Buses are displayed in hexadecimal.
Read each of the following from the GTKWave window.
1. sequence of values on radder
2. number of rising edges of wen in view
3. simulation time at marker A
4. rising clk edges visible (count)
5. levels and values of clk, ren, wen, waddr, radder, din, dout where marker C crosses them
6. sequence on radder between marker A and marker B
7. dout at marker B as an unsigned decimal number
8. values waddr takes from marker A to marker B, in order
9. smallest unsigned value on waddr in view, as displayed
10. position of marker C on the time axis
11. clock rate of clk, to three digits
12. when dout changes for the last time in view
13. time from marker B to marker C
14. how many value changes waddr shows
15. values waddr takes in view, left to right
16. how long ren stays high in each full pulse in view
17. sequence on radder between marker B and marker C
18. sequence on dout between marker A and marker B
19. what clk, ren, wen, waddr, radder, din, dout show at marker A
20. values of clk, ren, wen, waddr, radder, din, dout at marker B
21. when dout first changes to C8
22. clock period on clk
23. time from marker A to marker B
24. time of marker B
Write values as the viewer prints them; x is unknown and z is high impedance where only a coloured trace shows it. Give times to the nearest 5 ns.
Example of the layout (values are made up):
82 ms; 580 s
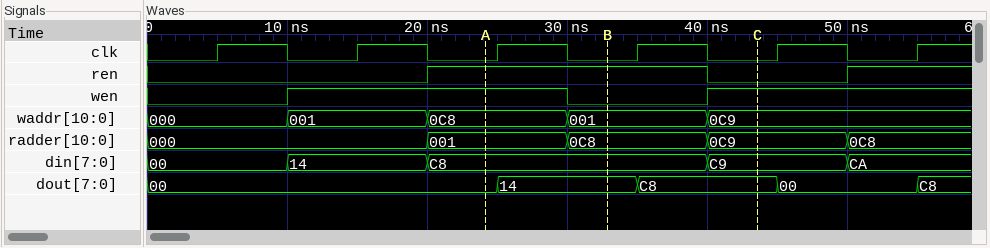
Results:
000, 001, 0C8, 0C9, 0C8; 2; 25 ns; 6; clk=0, ren=0, wen=1, waddr=0C9, radder=0C9, din=C9, dout=C8; 001, 0C8; 20; 0C8, 001; 000; 45 ns; 100 MHz; 55 ns; 10 ns; 4; 000, 001, 0C8, 001, 0C9; 20 ns; 0C8, 0C9; 00, 14; clk=0, ren=1, wen=1, waddr=0C8, radder=001, din=C8, dout=00; clk=0, ren=1, wen=0, waddr=001, radder=0C8, din=C8, dout=14; 35 ns; 10 ns; 10 ns; 35 ns
